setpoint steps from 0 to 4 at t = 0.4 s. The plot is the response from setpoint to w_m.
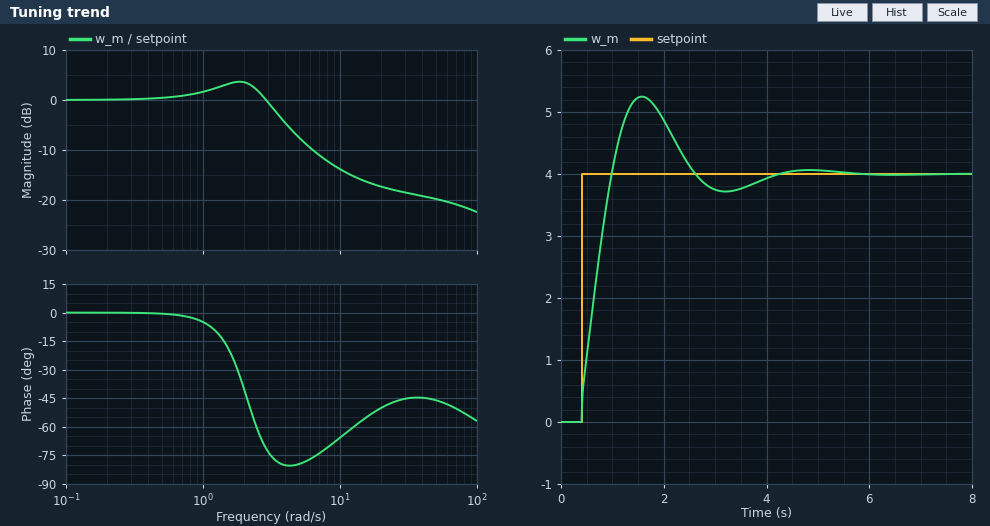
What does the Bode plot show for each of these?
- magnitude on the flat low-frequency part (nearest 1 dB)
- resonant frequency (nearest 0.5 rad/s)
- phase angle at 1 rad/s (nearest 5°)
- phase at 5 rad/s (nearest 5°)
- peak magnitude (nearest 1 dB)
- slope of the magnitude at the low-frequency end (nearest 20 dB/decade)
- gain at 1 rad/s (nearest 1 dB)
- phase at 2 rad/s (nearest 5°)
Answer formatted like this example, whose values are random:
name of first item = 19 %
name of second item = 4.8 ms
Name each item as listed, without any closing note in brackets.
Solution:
magnitude on the flat low-frequency part = 0 dB
resonant frequency = 2.0 rad/s
phase angle at 1 rad/s = -5°
phase at 5 rad/s = -80°
peak magnitude = 4 dB
slope of the magnitude at the low-frequency end = 0 dB/decade
gain at 1 rad/s = 2 dB
phase at 2 rad/s = -40°
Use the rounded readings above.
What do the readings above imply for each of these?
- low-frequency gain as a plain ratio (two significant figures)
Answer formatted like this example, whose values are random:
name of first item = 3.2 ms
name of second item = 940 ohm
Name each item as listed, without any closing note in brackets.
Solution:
low-frequency gain as a plain ratio = 1.0
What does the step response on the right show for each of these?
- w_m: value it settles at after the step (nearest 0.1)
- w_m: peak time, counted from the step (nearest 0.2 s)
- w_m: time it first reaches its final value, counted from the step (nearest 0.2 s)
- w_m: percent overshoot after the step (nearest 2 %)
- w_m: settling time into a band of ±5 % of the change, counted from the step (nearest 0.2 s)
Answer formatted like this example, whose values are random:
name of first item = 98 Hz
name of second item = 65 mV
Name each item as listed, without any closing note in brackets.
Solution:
w_m: value it settles at after the step = 4.0
w_m: peak time, counted from the step = 1.2 s
w_m: time it first reaches its final value, counted from the step = 0.6 s
w_m: percent overshoot after the step = 32 %
w_m: settling time into a band of ±5 % of the change, counted from the step = 3.2 s
